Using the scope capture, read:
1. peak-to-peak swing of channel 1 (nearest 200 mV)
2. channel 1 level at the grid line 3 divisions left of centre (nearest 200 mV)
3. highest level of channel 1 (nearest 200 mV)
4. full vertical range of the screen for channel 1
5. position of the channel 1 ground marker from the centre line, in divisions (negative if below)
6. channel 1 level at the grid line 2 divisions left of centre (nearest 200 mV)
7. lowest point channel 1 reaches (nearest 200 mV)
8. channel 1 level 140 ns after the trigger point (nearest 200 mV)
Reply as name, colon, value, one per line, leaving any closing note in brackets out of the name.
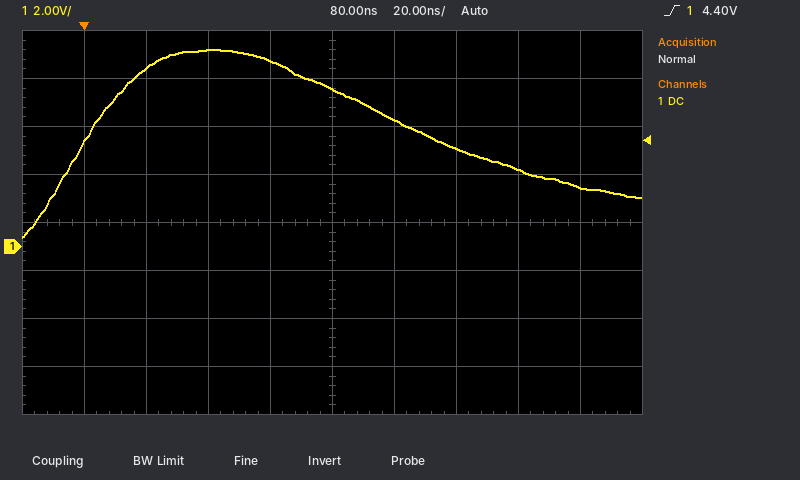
peak-to-peak swing of channel 1: 7.8 V
channel 1 level at the grid line 3 divisions left of centre: 7.4 V
highest level of channel 1: 8.2 V
full vertical range of the screen for channel 1: 16 V
position of the channel 1 ground marker from the centre line, in divisions: -0.5 div
channel 1 level at the grid line 2 divisions left of centre: 8.2 V
lowest point channel 1 reaches: 400 mV
channel 1 level 140 ns after the trigger point: 3.2 V
